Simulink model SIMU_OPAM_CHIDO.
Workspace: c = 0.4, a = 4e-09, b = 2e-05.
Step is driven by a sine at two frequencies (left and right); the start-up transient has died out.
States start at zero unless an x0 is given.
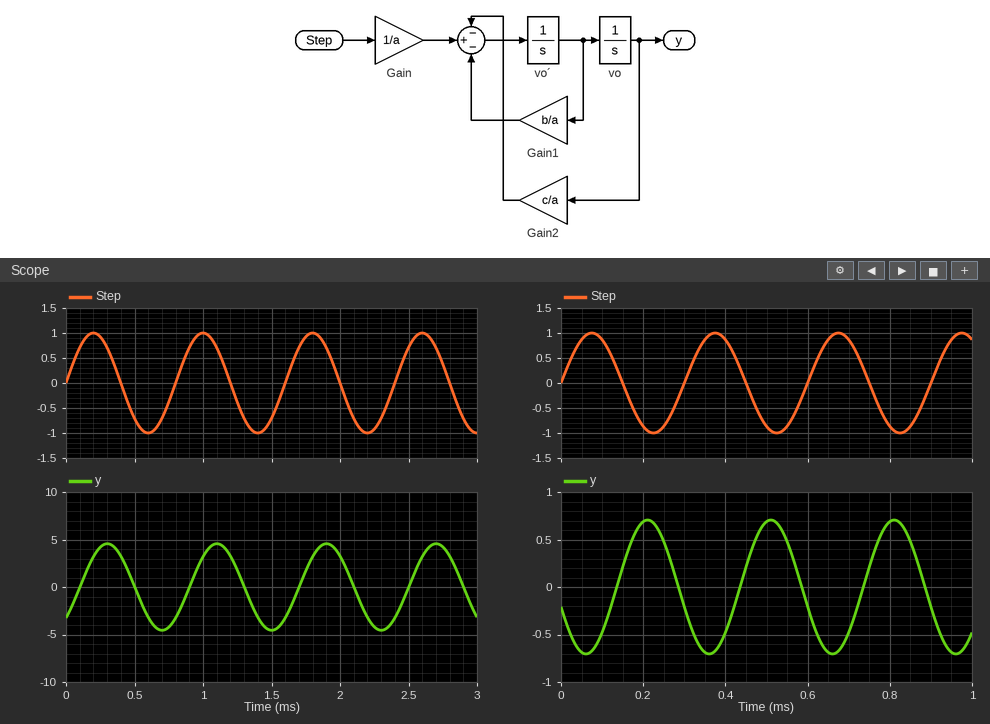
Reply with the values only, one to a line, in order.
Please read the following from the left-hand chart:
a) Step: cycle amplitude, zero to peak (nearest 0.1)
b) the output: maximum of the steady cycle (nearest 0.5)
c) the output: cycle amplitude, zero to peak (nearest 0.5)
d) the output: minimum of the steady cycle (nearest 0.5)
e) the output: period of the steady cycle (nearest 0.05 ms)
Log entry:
1.0
4.5
4.5
-4.5
0.80 ms
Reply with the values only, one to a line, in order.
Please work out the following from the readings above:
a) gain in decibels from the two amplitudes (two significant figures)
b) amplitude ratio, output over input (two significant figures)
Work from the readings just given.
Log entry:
13 dB
4.5
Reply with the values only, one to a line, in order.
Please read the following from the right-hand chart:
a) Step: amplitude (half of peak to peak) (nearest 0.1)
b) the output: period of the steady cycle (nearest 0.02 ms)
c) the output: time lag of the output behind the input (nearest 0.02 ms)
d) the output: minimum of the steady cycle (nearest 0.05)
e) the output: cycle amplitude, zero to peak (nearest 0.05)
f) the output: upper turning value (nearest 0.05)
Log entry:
1.0
0.30 ms
0.14 ms
-0.70
0.70
0.70
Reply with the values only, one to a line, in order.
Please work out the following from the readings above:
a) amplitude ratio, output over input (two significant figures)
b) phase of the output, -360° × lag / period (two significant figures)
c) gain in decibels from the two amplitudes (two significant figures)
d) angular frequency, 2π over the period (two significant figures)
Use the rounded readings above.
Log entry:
0.70
-170°
-3.1 dB
21 rad/ms
